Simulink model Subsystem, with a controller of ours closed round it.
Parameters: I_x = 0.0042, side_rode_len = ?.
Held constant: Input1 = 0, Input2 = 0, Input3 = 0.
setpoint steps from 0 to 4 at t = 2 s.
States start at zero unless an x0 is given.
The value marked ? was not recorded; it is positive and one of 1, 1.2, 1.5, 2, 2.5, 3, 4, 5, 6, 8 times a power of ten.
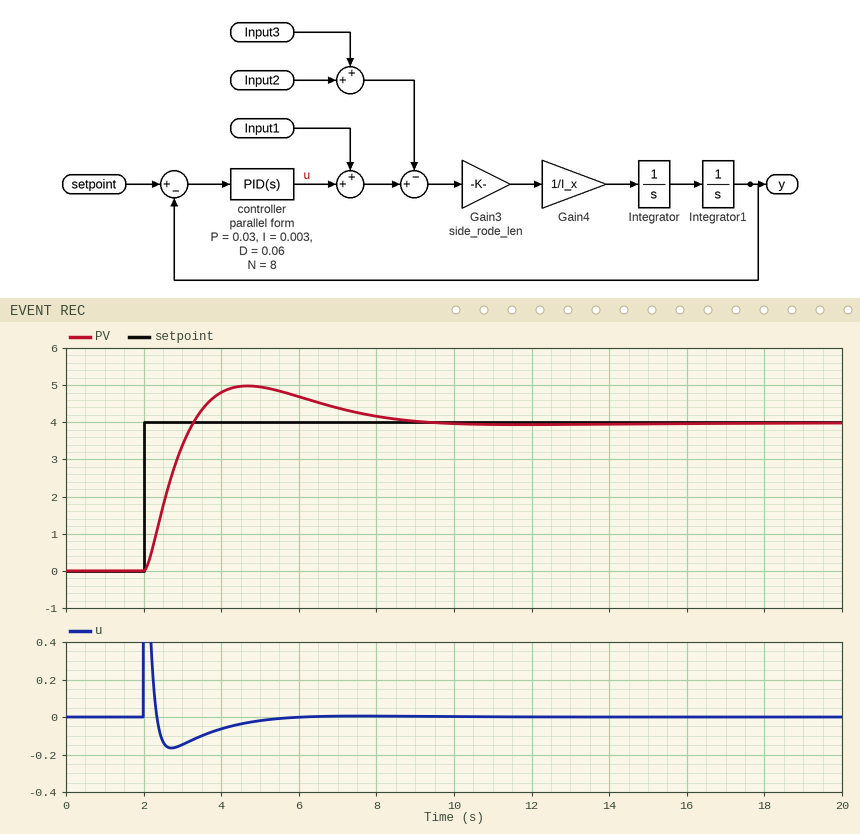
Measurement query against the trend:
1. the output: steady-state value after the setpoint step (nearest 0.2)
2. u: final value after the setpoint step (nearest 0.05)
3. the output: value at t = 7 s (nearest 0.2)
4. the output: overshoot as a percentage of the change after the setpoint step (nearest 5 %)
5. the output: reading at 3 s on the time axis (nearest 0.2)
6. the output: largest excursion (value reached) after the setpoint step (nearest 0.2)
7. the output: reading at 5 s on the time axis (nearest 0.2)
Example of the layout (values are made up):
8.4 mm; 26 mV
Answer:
4.0; 0.00; 4.4; 25 %; 3.4; 5.0; 5.0
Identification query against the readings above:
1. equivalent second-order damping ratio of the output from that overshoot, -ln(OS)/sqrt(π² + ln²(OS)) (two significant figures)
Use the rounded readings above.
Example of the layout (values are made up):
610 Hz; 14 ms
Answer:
0.40
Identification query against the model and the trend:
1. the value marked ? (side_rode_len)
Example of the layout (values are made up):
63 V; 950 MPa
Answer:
0.08
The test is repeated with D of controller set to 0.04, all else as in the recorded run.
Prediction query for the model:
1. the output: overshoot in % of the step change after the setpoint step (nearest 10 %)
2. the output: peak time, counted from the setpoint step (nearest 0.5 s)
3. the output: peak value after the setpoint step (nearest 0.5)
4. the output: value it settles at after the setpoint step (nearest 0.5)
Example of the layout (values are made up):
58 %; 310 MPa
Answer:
40 %; 3.0 s; 5.5; 4.0
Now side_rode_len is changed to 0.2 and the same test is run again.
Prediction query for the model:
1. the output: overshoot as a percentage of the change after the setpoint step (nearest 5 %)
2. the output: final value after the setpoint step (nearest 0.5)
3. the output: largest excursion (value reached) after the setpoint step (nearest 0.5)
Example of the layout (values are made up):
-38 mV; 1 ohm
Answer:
15 %; 4.0; 4.5
